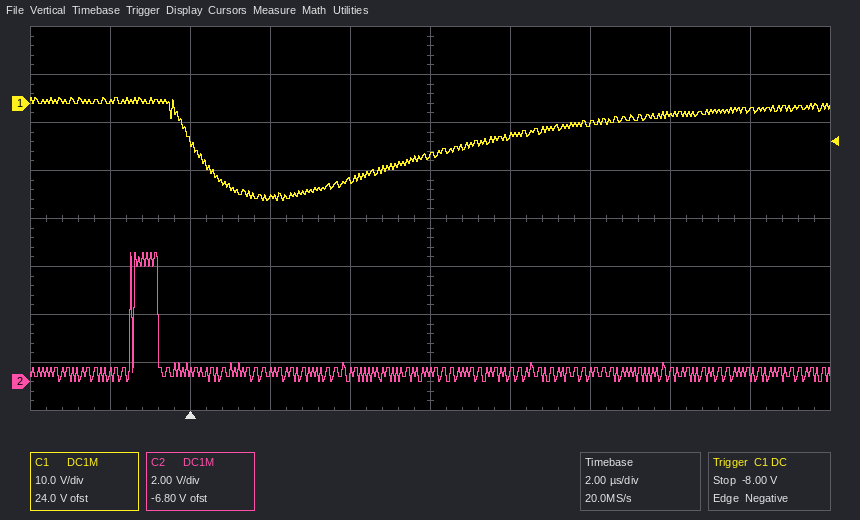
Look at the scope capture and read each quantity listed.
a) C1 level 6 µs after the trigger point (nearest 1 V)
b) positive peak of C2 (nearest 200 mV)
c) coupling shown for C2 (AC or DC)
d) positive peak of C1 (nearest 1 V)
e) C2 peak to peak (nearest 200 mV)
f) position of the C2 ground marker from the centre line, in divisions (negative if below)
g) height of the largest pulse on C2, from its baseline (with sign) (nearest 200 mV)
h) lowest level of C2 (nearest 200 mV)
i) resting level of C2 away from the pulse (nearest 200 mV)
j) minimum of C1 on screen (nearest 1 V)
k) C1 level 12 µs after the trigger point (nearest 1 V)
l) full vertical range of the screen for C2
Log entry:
-11 V
5.4 V
DC
1 V
5.4 V
-3.4 div
+5.0 V
0.0 V
400 mV
-20 V
-2 V
16 V
